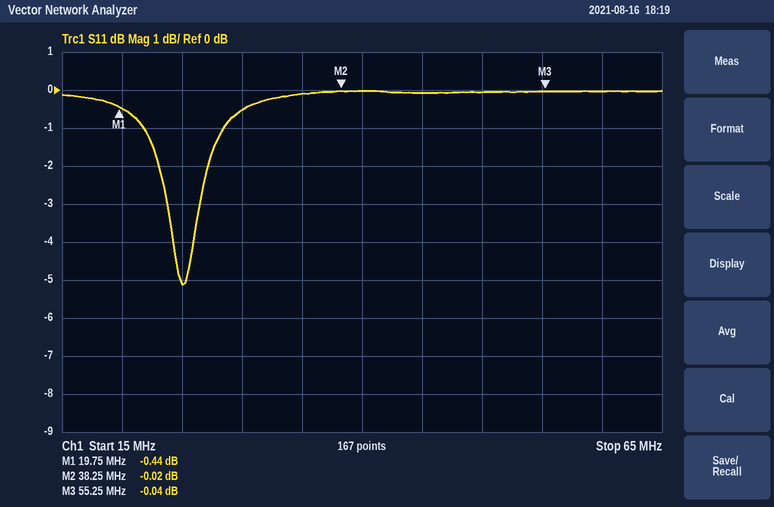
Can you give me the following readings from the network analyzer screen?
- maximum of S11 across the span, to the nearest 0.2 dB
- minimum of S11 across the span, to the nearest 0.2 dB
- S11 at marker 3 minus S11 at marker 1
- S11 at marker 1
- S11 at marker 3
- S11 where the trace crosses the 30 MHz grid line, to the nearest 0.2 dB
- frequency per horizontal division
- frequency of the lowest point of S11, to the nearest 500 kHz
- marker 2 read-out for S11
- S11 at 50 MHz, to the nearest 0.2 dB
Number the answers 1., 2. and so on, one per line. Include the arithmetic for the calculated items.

1. 0.0 dB
2. -5.2 dB
3. -0.04 − (-0.44) = 0.40 dB
4. -0.44 dB
5. -0.04 dB
6. -0.6 dB
7. 5 MHz
8. 25.0 MHz
9. -0.02 dB
10. 0.0 dB
